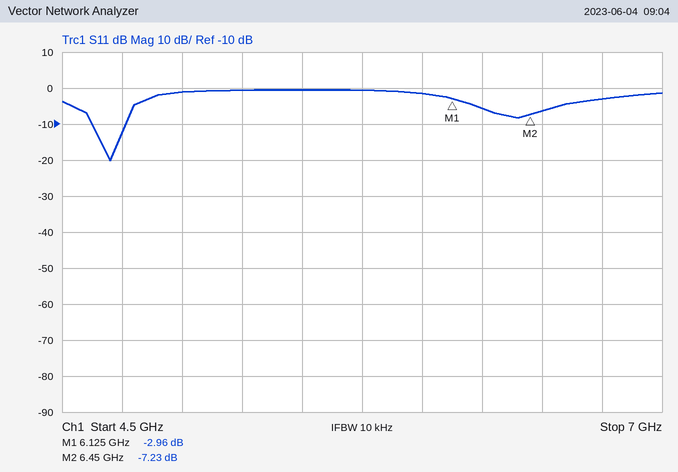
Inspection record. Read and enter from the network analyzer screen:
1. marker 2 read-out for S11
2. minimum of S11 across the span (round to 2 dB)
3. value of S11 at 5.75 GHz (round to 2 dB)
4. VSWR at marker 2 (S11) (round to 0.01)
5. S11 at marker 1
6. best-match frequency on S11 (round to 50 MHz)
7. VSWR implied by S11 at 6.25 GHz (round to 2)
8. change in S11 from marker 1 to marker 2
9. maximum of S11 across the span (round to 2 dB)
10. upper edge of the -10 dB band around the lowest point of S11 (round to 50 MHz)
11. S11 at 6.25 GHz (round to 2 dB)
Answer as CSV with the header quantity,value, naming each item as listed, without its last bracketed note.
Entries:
quantity,value
marker 2 read-out for S11,-7.23 dB
minimum of S11 across the span,-20 dB
value of S11 at 5.75 GHz,0 dB
VSWR at marker 2 (S11),2.54
S11 at marker 1,-2.96 dB
best-match frequency on S11,4.70 GHz
VSWR implied by S11 at 6.25 GHz,4
change in S11 from marker 1 to marker 2,-4.27 dB
maximum of S11 across the span,0 dB
upper edge of the -10 dB band around the lowest point of S11,4.75 GHz
S11 at 6.25 GHz,-6 dB
